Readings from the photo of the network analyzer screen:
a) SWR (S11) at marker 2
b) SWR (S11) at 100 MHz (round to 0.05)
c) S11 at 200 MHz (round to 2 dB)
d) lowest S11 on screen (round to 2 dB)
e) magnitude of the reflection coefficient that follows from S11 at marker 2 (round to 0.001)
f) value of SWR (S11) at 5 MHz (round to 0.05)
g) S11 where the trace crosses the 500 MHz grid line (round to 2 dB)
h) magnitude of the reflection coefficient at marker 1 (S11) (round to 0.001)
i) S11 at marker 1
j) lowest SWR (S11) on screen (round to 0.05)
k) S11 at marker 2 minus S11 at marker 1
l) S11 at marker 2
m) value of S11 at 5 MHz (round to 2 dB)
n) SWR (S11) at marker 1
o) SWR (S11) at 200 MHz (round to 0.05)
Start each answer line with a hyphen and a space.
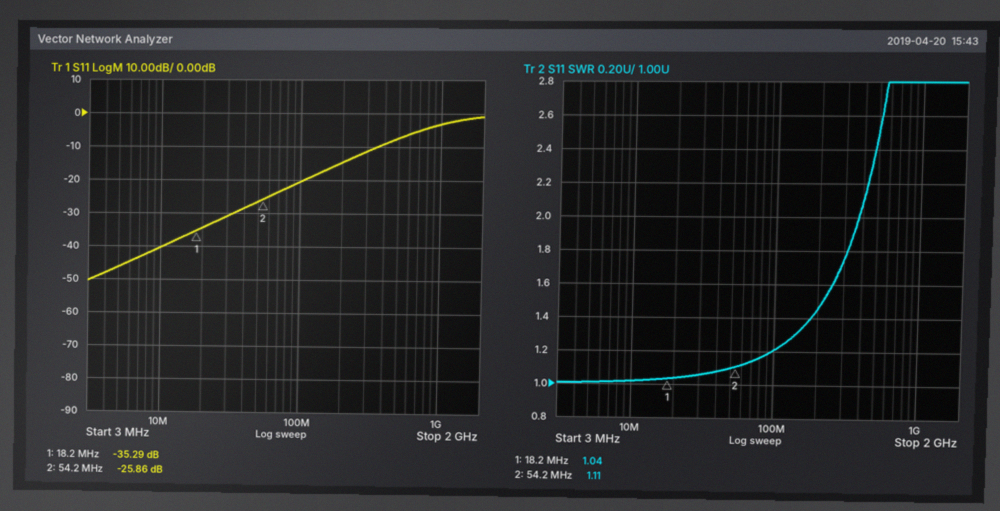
- 1.11
- 1.20
- -14 dB
- -50 dB
- 0.051
- 1.00
- -8 dB
- 0.017
- -35.29 dB
- 1.00
- 9.43 dB
- -25.86 dB
- -46 dB
- 1.04
- 1.45
